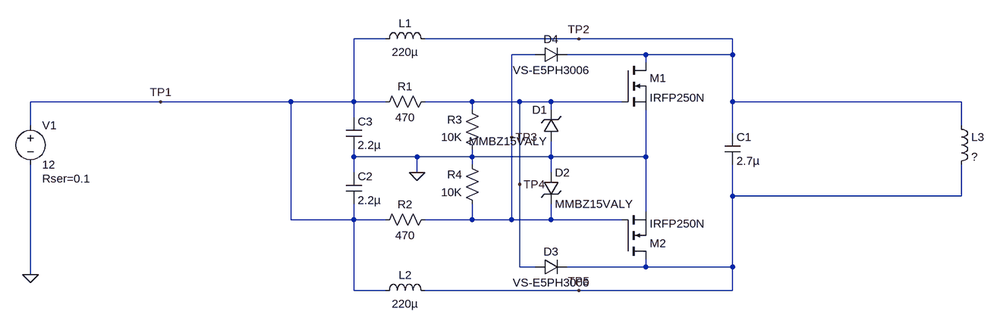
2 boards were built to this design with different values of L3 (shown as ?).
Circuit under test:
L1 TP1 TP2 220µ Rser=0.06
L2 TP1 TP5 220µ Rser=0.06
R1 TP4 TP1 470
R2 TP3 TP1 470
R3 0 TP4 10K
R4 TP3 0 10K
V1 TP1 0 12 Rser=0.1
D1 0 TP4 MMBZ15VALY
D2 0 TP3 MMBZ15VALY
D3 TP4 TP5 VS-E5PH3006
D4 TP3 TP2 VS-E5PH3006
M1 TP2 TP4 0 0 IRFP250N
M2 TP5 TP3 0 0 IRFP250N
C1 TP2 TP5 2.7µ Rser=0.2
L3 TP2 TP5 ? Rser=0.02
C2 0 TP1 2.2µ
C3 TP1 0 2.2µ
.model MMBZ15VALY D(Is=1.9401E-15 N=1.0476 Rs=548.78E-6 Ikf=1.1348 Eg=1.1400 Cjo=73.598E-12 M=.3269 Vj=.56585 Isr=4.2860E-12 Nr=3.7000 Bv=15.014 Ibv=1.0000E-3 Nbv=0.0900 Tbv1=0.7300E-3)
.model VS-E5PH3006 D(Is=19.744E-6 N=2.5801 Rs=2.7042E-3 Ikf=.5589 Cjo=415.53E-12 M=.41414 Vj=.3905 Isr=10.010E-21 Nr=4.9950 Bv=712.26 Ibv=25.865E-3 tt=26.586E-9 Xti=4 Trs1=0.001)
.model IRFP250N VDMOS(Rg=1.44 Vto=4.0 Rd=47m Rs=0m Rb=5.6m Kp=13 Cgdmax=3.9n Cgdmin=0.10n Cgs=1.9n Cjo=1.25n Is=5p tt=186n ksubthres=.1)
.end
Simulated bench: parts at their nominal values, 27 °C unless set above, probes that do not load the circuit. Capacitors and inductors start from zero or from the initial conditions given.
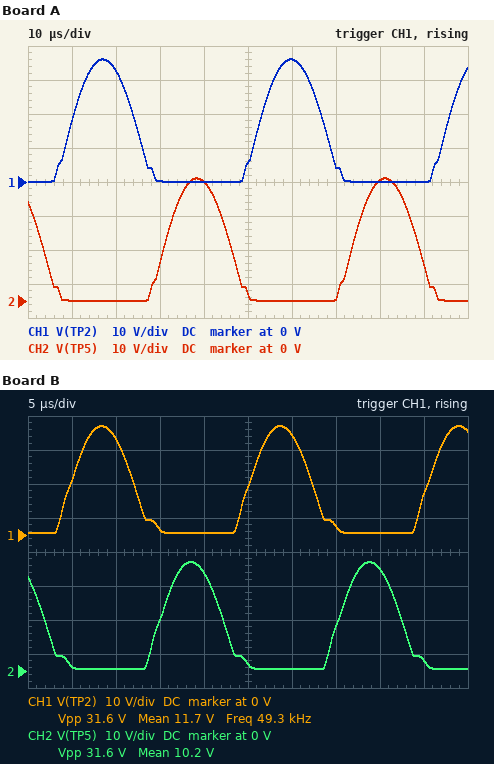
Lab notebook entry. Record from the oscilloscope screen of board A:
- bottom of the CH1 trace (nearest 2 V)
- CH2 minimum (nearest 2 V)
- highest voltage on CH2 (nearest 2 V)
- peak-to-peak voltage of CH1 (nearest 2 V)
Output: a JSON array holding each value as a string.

["0 V", "0 V", "36 V", "36 V"]
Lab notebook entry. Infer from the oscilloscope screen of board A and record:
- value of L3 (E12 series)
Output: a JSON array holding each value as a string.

["18 µH"]
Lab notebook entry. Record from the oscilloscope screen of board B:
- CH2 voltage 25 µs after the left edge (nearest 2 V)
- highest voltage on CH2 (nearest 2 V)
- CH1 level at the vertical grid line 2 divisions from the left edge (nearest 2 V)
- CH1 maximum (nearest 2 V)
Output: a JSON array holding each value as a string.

["2 V", "32 V", "28 V", "32 V"]
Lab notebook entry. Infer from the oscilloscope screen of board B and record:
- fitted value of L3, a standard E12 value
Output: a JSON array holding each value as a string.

["3.9 µH"]
